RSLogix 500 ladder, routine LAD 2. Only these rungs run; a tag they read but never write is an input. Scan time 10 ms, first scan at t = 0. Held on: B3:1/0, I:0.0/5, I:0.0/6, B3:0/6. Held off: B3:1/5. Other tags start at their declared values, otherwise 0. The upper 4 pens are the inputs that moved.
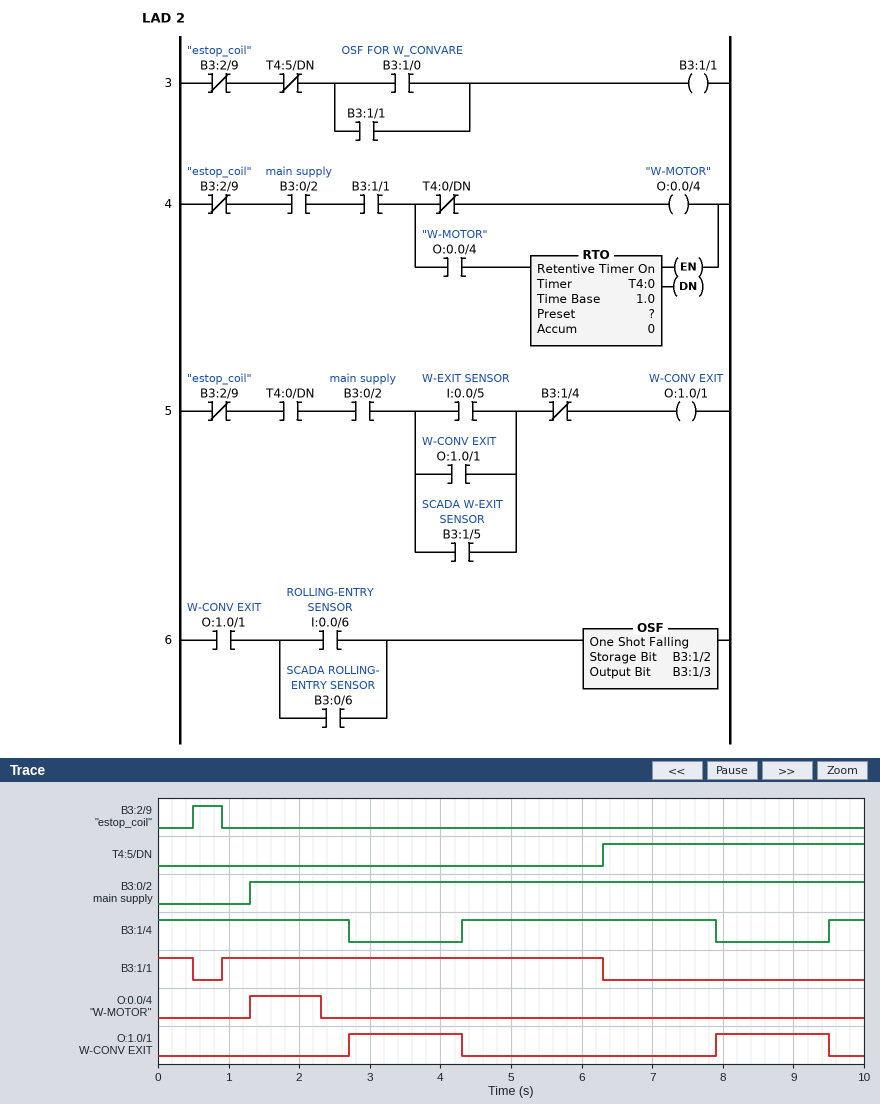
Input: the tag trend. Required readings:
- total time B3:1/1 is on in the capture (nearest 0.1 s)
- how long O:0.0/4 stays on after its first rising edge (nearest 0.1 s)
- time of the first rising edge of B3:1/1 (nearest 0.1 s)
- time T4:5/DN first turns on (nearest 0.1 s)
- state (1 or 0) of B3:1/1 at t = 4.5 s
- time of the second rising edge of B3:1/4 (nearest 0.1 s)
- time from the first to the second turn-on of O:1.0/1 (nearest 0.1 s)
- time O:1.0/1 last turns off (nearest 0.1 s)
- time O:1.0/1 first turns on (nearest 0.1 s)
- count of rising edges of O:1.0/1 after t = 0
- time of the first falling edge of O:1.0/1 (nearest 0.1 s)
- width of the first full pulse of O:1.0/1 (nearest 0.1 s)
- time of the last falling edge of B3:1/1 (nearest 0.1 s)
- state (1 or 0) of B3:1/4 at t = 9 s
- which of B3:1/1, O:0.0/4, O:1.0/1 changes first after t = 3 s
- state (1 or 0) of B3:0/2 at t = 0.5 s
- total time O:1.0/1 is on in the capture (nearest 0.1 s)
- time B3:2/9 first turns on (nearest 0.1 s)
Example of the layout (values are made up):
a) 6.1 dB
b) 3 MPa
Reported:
a) 5.9 s
b) 1.0 s
c) 0.9 s
d) 6.3 s
e) 1
f) 9.5 s
g) 5.2 s
h) 9.5 s
i) 2.7 s
j) 2
k) 4.3 s
l) 1.6 s
m) 6.3 s
n) 0
o) O:1.0/1
p) 0
q) 3.2 s
r) 0.5 s
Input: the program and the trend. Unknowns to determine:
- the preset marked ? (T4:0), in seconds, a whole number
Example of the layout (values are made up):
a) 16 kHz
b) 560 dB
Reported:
a) 1 s
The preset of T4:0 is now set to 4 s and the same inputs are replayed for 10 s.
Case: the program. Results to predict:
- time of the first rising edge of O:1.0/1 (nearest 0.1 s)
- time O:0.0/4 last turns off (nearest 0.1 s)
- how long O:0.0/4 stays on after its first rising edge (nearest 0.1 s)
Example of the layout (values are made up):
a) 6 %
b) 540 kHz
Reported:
a) 7.9 s
b) 5.3 s
c) 4.0 s
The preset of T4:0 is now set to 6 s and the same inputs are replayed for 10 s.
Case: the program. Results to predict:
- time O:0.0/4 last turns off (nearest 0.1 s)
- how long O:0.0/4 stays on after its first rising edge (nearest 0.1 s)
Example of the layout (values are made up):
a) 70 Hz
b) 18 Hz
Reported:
a) 6.3 s
b) 5.0 s
